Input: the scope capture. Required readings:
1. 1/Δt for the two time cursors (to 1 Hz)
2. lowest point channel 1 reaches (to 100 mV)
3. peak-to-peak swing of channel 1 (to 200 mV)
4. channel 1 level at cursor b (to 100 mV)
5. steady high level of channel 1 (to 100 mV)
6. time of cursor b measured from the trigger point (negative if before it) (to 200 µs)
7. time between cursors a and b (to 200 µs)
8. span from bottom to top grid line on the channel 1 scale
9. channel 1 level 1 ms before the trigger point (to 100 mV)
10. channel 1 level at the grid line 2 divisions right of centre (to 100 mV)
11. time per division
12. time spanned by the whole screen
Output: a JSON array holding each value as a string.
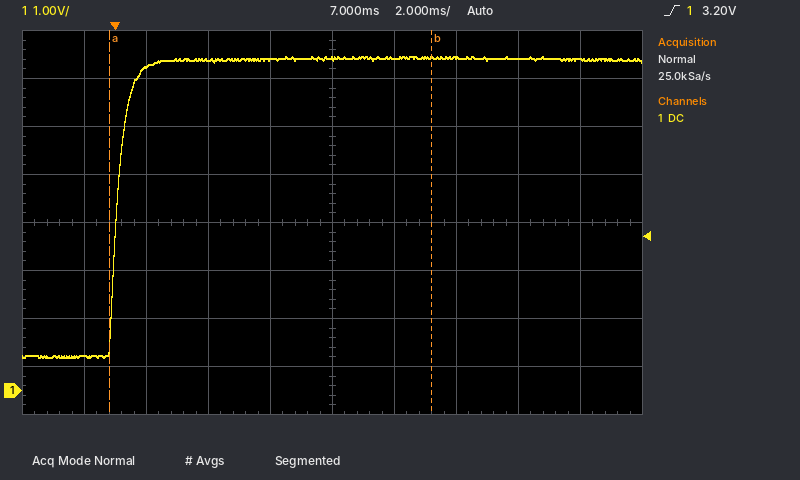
["96 Hz", "700 mV", "6.2 V", "6.9 V", "6.9 V", "+10.2 ms", "10.4 ms", "8 V", "700 mV", "6.9 V", "2 ms", "20 ms"]
